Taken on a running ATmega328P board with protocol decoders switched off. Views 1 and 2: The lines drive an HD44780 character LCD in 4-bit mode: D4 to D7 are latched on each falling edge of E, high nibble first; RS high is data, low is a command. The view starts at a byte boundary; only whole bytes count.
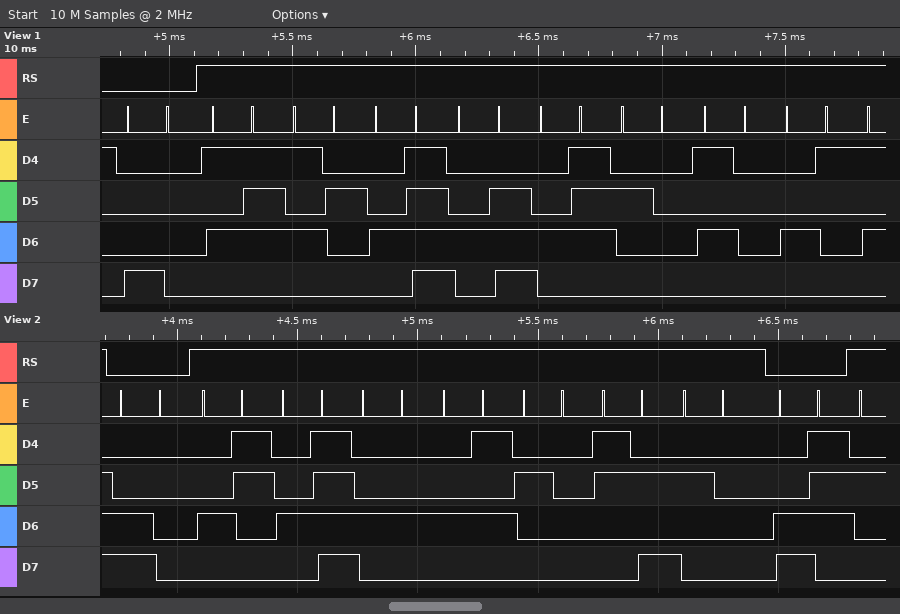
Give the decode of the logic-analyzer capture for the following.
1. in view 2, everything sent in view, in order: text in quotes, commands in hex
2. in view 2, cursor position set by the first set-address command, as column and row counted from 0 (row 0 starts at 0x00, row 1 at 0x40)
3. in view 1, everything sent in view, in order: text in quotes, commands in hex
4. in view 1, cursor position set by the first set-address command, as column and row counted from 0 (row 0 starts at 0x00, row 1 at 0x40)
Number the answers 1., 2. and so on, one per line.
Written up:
1. 0xC0 "CODE : " 0xC7
2. column 0, row 1
3. 0x80 "WRONG PA"
4. column 0, row 0
